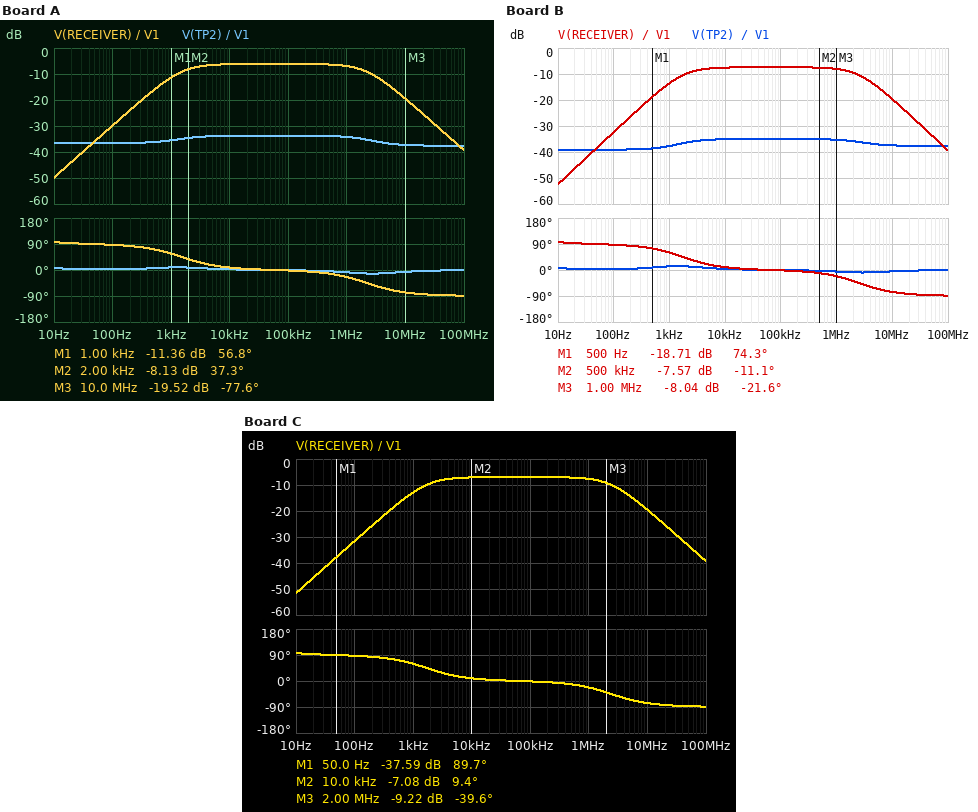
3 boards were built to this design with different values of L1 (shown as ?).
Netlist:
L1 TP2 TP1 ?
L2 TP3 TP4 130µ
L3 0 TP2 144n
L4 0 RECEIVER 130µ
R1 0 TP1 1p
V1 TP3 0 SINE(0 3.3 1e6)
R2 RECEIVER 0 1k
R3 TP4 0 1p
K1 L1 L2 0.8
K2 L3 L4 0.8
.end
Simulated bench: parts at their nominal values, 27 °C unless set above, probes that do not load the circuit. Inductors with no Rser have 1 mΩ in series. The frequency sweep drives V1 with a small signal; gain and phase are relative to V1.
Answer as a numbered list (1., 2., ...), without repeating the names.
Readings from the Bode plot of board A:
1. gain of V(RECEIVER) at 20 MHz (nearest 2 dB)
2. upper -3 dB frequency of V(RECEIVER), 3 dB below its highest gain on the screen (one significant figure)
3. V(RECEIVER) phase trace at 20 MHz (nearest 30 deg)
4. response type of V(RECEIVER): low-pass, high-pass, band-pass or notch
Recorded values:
1. -26 dB
2. 2 MHz
3. -90 deg
4. band-pass
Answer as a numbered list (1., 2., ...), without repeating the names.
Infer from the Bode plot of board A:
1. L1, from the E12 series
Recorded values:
1. 180 nH
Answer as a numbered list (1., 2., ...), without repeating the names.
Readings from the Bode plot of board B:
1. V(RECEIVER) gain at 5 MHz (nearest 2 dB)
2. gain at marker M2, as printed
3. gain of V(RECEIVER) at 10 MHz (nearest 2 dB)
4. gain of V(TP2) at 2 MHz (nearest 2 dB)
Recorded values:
1. -14 dB
2. -7.57 dB
3. -20 dB
4. -36 dB
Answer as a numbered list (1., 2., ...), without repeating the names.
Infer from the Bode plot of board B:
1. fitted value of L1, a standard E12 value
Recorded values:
1. 100 nH
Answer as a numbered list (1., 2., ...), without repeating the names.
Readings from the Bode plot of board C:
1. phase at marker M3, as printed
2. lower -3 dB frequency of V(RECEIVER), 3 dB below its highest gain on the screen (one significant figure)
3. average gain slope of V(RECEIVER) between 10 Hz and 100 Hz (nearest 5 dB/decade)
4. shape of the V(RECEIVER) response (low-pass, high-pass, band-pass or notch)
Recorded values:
1. -39.6 deg
2. 2 kHz
3. 20 dB/decade
4. band-pass
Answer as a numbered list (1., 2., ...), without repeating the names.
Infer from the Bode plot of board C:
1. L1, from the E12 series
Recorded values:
1. 120 nH
